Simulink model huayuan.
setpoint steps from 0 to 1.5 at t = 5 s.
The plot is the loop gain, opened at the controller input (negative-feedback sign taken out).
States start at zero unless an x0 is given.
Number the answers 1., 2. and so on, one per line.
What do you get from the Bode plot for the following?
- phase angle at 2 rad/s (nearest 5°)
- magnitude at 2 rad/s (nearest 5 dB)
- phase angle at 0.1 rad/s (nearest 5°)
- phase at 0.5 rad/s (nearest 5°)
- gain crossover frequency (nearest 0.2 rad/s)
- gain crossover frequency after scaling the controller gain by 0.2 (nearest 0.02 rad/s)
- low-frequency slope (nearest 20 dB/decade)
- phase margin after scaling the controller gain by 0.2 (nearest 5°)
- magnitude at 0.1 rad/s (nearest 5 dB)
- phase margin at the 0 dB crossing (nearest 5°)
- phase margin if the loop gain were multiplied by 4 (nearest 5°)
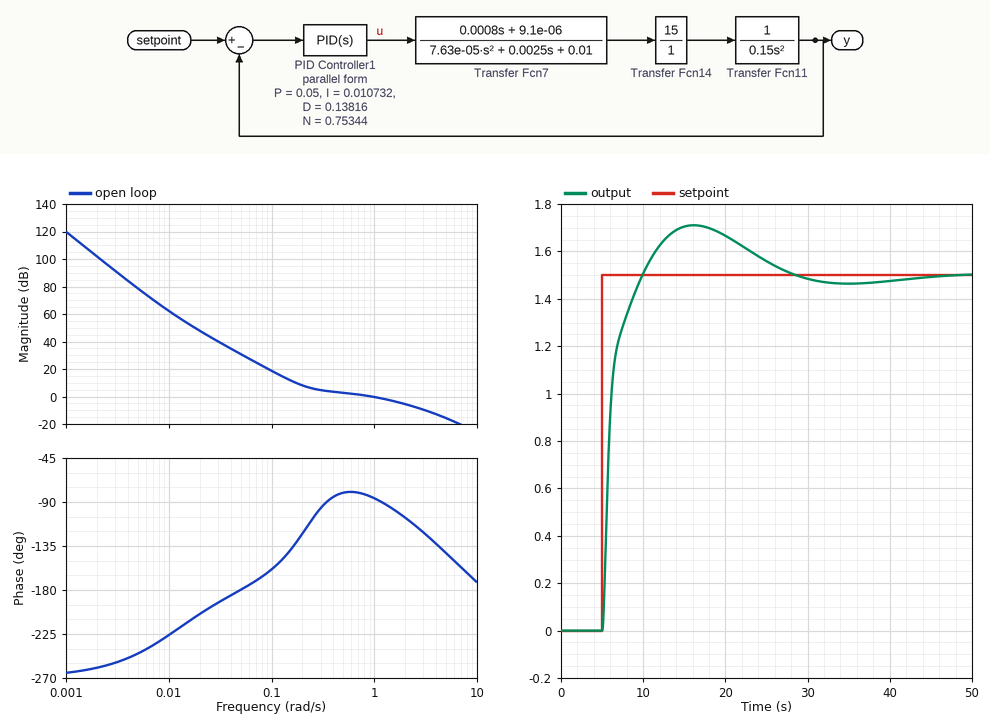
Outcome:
1. -105°
2. -5 dB
3. -160°
4. -80°
5. 1.0 rad/s
6. 0.14 rad/s
7. -60 dB/decade
8. 35°
9. 20 dB
10. 95°
11. 50°
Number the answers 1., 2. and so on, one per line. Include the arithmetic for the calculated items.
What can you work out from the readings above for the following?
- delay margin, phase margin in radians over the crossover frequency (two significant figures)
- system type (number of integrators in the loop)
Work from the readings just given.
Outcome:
1. 95 × π / 180 / 1 = 1.7 s
2. 3
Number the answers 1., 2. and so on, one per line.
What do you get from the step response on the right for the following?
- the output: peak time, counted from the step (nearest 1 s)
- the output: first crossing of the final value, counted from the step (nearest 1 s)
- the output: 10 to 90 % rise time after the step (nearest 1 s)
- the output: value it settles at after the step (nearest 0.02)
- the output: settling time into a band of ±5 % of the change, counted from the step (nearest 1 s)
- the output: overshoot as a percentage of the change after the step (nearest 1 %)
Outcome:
1. 11 s
2. 5 s
3. 3 s
4. 1.50
5. 19 s
6. 14 %
